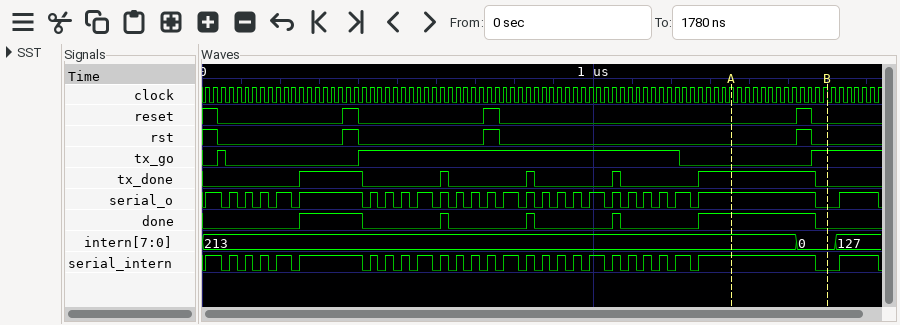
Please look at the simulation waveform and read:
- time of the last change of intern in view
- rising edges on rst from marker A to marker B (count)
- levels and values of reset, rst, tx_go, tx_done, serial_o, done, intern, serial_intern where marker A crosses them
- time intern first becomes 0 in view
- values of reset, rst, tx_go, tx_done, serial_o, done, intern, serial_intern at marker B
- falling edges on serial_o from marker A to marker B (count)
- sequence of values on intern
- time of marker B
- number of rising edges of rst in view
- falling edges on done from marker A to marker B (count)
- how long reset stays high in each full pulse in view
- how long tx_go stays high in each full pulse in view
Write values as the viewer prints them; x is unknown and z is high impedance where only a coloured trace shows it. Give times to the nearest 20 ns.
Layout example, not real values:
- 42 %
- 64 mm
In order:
- 1620 ns
- 1
- reset=0, rst=0, tx_go=0, tx_done=1, serial_o=1, done=1, intern=213, serial_intern=1
- 1520 ns
- reset=0, rst=0, tx_go=1, tx_done=0, serial_o=0, done=0, intern=0, serial_intern=0
- 1
- 213, 0, 127
- 1600 ns
- 3
- 1
- 40 ns, 40 ns, 40 ns
- 20 ns, 820 ns
